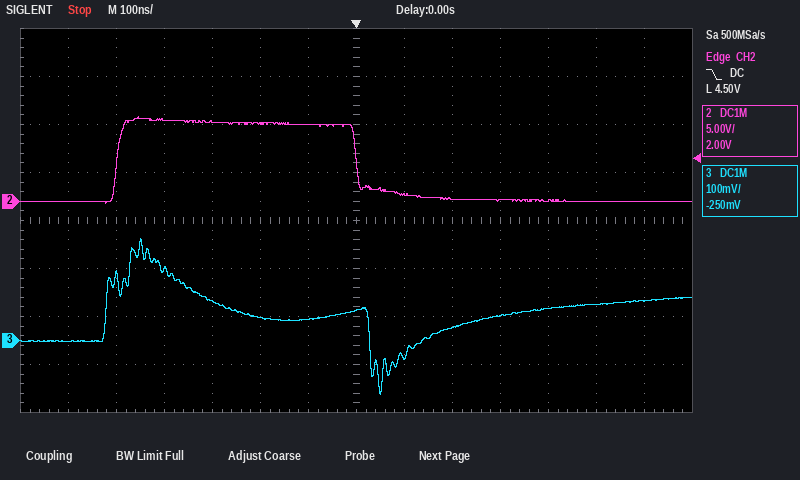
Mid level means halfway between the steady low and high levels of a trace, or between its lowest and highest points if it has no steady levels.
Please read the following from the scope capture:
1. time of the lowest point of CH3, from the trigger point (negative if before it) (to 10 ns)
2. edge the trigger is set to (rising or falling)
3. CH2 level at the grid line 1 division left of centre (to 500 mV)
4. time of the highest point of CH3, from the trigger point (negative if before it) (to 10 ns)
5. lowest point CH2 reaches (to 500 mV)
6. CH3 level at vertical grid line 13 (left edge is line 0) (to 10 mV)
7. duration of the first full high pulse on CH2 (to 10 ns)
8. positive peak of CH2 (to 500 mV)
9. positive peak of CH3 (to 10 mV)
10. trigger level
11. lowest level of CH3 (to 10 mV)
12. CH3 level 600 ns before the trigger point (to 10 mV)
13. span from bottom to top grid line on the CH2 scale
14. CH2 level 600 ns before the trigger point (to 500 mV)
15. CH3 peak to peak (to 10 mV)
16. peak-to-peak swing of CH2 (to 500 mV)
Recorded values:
+50 ns
falling
8.0 V
-450 ns
0.0 V
80 mV
500 ns
9.0 V
210 mV
4.50 V
-110 mV
0 mV
40 V
0.0 V
320 mV
9.0 V
